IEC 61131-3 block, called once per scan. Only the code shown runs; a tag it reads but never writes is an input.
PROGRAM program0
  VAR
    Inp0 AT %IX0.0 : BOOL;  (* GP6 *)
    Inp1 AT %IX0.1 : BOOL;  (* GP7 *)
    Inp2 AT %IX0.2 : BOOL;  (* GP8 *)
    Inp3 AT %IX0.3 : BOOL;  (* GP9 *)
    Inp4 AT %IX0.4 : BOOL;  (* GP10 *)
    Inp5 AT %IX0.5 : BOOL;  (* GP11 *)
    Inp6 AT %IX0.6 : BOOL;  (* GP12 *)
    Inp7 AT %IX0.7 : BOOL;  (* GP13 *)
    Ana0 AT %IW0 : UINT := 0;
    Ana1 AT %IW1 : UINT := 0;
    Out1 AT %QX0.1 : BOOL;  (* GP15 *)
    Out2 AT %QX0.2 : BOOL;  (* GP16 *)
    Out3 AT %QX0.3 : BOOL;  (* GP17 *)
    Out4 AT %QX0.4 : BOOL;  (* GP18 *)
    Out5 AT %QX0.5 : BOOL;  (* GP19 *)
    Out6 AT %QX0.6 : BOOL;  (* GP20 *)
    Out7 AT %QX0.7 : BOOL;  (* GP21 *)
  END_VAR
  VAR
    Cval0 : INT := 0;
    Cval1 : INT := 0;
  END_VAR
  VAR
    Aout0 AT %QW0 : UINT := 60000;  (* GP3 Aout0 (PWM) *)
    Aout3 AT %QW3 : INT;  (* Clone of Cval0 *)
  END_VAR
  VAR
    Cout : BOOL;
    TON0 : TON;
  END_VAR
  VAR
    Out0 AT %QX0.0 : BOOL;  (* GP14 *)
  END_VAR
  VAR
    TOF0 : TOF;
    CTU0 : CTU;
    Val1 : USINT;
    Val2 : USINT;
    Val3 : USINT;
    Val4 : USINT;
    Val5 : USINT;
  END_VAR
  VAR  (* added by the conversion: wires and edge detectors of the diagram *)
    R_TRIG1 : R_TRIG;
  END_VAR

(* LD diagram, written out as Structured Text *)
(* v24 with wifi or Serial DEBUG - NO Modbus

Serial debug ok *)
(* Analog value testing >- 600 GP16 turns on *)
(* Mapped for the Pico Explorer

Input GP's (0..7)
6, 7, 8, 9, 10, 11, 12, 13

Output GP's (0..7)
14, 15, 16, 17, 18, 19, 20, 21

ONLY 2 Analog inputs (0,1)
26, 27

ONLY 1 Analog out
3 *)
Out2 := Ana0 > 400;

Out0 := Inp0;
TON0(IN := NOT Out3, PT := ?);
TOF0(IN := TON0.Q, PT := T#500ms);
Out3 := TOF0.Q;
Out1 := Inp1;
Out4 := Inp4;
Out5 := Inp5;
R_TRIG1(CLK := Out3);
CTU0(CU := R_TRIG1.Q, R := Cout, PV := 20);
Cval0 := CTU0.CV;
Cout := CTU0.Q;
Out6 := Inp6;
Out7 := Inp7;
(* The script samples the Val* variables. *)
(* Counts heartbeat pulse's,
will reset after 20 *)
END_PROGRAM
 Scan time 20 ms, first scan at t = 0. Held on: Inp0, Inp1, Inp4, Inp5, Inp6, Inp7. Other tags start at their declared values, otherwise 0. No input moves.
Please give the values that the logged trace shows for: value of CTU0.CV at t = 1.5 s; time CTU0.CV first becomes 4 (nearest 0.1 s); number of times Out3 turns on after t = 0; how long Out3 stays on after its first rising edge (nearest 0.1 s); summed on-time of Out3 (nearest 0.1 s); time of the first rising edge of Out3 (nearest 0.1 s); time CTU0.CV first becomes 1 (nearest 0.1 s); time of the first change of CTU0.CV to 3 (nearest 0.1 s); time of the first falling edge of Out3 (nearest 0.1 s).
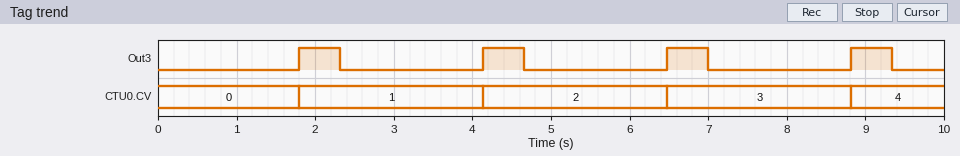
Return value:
0
8.8 s
4
0.5 s
2.1 s
1.8 s
1.8 s
6.5 s
2.3 s
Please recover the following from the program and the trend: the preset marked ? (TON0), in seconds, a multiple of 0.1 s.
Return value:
1.8 s
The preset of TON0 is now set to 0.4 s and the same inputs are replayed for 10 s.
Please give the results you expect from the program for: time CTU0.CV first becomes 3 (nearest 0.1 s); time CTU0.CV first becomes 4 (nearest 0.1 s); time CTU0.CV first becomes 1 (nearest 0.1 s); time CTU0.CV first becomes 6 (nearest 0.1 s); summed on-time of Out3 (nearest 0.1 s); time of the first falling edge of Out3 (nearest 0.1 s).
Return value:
2.3 s
3.2 s
0.4 s
5.1 s
5.4 s
0.9 s
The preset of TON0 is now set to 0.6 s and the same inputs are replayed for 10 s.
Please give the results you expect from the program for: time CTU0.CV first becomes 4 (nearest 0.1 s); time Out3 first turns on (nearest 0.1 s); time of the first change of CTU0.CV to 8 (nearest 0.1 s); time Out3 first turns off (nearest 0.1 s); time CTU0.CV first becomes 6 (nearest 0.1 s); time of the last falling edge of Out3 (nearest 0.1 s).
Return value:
4.0 s
0.6 s
8.6 s
1.1 s
6.3 s
9.1 s
